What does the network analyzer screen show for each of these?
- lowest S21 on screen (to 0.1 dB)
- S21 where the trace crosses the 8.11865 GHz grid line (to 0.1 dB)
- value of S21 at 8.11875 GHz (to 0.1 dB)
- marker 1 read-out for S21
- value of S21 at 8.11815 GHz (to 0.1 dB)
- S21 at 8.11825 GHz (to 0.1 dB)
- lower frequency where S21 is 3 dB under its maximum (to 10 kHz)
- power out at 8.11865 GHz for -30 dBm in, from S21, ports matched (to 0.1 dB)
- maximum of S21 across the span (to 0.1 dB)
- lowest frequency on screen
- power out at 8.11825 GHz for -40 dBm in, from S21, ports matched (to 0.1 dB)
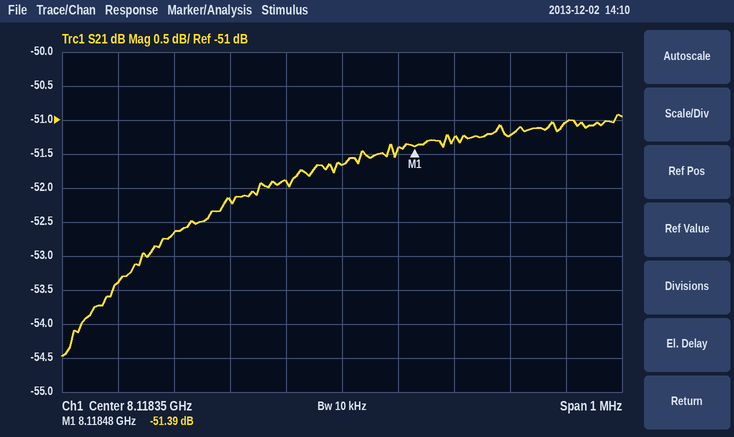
-54.5 dB
-51.2 dB
-51.0 dB
-51.39 dB
-52.2 dB
-51.9 dB
8.11789 GHz
-81.2 dBm
-50.9 dB
8.11785 GHz
-91.9 dBm
